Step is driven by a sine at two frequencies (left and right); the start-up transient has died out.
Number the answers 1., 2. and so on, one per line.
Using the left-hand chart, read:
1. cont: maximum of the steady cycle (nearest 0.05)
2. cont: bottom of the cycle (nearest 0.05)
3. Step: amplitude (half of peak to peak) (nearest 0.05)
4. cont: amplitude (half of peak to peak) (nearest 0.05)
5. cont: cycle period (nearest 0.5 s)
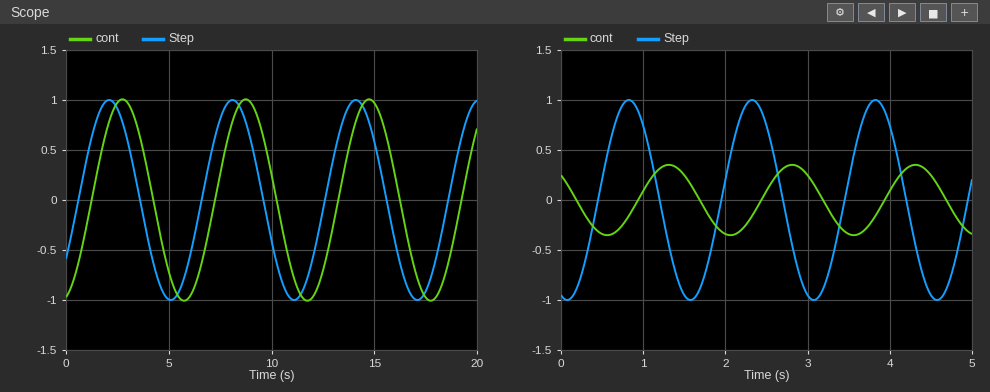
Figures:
1. 1.00
2. -1.00
3. 1.00
4. 1.00
5. 6.0 s
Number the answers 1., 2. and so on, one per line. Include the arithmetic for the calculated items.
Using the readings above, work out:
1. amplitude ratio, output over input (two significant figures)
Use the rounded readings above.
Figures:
1. 1 / 1 = 1.0
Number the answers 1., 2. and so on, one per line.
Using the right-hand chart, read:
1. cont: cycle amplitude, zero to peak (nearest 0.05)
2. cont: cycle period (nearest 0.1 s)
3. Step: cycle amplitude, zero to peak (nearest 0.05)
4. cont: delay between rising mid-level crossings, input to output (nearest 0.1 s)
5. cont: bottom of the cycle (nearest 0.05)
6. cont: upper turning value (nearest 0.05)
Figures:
1. 0.35
2. 1.5 s
3. 1.00
4. 0.5 s
5. -0.35
6. 0.35
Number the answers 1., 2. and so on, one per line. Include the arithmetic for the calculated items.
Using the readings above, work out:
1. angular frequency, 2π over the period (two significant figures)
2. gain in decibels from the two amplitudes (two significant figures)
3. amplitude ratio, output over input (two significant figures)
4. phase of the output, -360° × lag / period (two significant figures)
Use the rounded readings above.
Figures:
1. 2π / 1.5 = 4.2 rad/s
2. 20 log10(0.35 / 1) = -9.1 dB
3. 0.35 / 1 = 0.35
4. -360 × 0.5 / 1.5 = -120°
